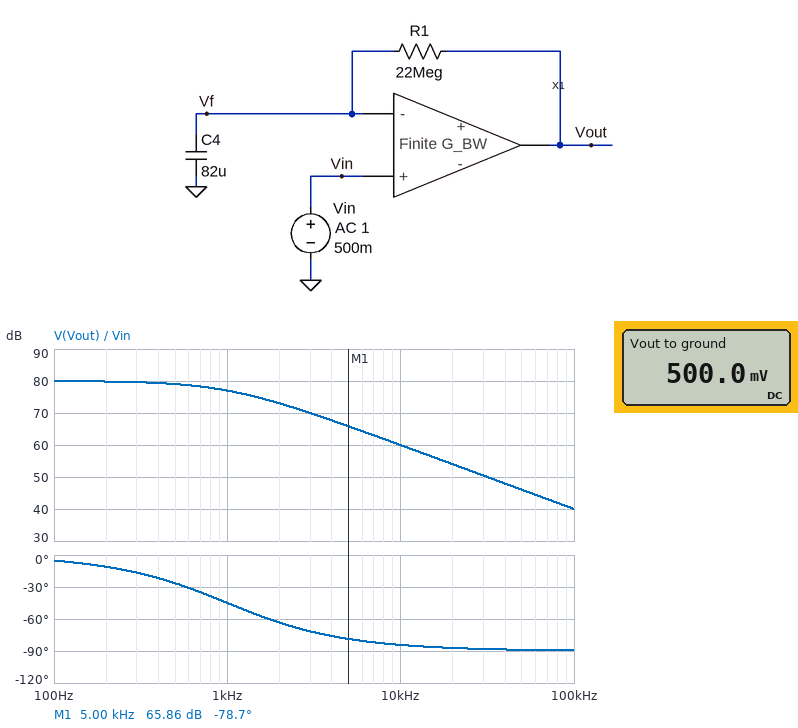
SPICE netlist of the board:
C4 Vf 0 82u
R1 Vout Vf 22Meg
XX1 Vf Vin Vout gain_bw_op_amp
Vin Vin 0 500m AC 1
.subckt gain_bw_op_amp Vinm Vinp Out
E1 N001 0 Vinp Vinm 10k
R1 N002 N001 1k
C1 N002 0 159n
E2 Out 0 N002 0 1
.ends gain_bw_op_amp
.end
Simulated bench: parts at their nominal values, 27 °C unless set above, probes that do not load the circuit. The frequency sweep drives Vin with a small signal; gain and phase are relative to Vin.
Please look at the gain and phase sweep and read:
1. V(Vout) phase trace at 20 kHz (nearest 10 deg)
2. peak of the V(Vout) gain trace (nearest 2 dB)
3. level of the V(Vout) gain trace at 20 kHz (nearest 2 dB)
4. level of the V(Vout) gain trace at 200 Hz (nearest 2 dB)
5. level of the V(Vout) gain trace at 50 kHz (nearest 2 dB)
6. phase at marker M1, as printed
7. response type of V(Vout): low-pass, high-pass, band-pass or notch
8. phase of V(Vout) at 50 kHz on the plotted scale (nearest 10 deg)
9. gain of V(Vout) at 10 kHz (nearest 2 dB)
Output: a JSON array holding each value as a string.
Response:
["-90 deg", "80 dB", "54 dB", "80 dB", "46 dB", "-78.7 deg", "low-pass", "-90 deg", "60 dB"]
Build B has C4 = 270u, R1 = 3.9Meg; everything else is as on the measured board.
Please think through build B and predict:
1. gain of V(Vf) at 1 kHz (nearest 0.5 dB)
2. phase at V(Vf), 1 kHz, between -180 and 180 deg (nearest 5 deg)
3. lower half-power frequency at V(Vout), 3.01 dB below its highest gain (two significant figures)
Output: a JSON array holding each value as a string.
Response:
["-59.5 dB", "-135 deg", "1.5 Hz"]
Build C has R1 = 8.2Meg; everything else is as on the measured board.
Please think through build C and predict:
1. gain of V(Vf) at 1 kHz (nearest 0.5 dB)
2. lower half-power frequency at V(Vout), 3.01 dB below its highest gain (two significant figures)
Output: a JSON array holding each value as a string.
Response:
["-55.5 dB", "2.4 Hz"]
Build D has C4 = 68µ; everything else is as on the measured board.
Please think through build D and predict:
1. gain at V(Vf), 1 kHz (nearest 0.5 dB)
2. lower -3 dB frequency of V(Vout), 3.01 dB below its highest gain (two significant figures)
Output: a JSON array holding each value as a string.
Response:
["-62.5 dB", "1.1 Hz"]
